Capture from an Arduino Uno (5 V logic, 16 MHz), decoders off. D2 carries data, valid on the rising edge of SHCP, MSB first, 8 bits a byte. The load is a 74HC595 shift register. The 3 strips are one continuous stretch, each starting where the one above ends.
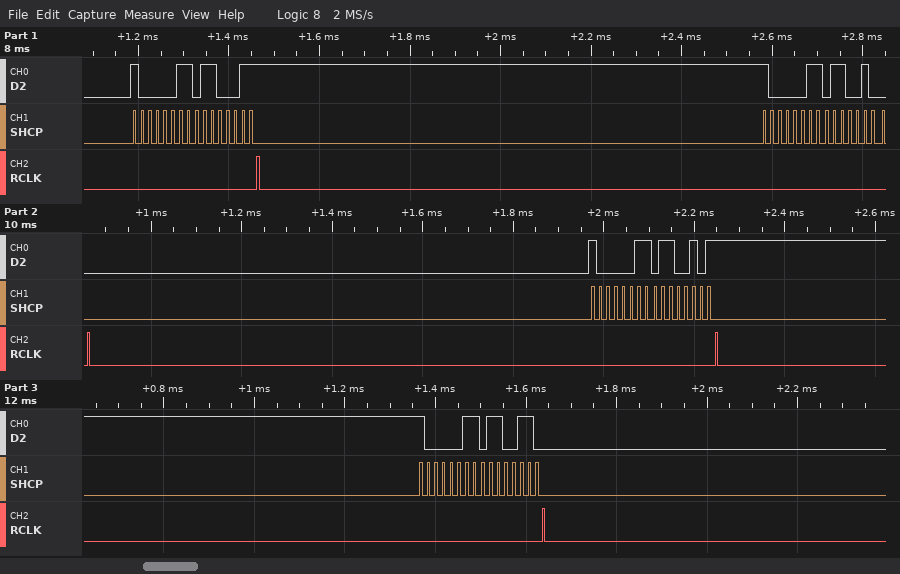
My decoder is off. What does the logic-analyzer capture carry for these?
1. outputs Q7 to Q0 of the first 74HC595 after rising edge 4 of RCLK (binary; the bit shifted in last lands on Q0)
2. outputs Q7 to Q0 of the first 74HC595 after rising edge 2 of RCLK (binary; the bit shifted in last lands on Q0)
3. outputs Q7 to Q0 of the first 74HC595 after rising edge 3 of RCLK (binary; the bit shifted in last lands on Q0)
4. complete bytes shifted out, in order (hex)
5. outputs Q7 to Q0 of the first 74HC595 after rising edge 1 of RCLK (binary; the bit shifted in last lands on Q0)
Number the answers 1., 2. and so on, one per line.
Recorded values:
1. 01100110
2. 01100100
3. 01100101
4. 83 63 83 64 83 65 83 66
5. 01100011
